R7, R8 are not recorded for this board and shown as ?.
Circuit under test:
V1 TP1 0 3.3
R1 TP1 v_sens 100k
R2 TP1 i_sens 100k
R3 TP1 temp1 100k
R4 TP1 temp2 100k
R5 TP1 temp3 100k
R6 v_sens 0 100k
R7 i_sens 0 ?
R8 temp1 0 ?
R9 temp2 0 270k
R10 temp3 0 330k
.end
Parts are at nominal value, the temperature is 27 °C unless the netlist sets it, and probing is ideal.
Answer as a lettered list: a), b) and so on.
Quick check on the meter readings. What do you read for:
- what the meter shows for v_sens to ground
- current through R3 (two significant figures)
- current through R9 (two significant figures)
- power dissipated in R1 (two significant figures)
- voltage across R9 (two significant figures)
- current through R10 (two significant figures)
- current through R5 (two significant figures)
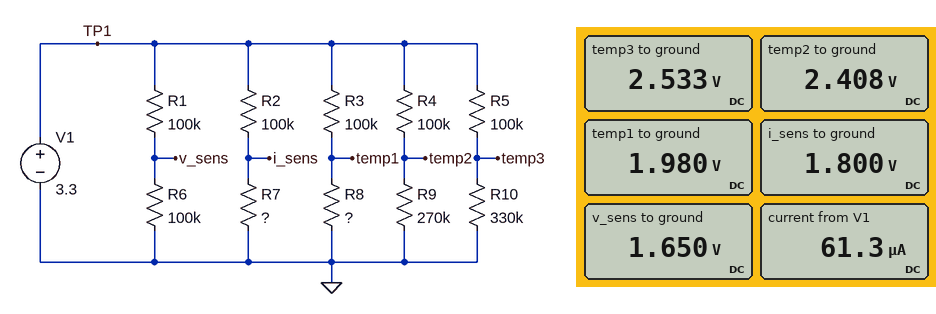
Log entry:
a) 1.650 V
b) 13 µA
c) 8.9 µA
d) 27 µW
e) 2.4 V
f) 7.7 µA
g) 7.7 µA
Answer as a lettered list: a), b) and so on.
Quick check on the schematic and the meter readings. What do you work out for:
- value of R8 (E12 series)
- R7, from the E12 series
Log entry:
a) 150 kΩ
b) 120 kΩ
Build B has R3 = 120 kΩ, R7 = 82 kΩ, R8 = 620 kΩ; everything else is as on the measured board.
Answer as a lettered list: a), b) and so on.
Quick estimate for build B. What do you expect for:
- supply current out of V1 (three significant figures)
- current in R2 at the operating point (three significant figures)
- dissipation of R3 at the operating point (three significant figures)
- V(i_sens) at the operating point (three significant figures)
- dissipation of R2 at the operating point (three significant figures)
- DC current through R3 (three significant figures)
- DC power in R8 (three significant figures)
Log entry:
a) 55.7 µA
b) 18.1 µA
c) 2.39 µW
d) 1.49 V
e) 32.9 µW
f) 4.46 µA
g) 12.3 µW
